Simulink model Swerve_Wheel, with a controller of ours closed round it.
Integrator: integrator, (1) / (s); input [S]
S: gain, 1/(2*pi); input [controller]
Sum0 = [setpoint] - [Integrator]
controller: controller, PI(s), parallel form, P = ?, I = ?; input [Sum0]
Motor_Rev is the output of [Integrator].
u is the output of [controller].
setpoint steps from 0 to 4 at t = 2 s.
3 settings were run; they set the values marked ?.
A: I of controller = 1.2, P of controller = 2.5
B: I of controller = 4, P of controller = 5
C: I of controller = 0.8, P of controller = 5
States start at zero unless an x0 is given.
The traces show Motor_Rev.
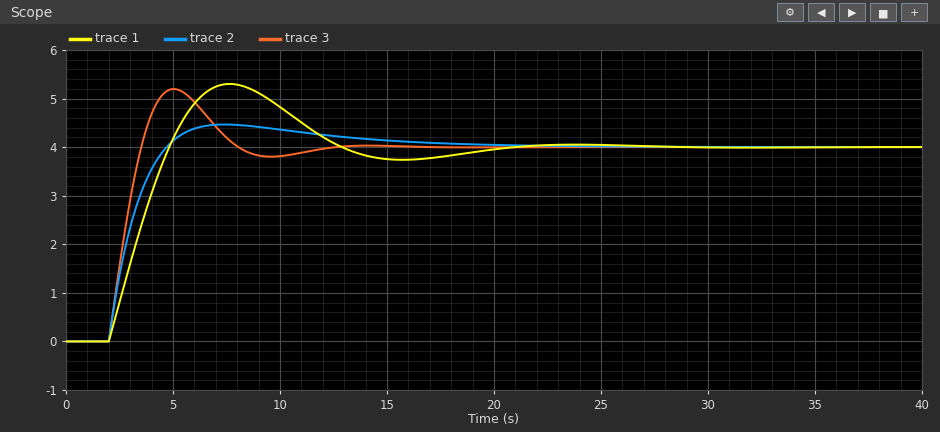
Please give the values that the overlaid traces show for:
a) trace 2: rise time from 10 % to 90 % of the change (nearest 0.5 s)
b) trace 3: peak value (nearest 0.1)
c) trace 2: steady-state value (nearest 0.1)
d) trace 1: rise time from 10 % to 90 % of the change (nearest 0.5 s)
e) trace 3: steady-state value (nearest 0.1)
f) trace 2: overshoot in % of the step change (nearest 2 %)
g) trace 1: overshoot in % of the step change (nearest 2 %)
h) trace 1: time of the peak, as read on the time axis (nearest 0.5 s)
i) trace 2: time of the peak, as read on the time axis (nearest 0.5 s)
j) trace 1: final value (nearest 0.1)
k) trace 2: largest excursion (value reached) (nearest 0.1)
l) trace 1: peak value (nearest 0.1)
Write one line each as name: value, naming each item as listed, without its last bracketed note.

trace 2: rise time from 10 % to 90 % of the change: 2.0 s
trace 3: peak value: 5.2
trace 2: steady-state value: 4.0
trace 1: rise time from 10 % to 90 % of the change: 2.0 s
trace 3: steady-state value: 4.0
trace 2: overshoot in % of the step change: 12 %
trace 1: overshoot in % of the step change: 32 %
trace 1: time of the peak, as read on the time axis: 7.5 s
trace 2: time of the peak, as read on the time axis: 7.5 s
trace 1: final value: 4.0
trace 2: largest excursion (value reached): 4.5
trace 1: peak value: 5.3
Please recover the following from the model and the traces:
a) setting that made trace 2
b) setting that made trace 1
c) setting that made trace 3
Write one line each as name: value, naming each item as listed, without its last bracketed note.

setting that made trace 2: C
setting that made trace 1: A
setting that made trace 3: B
